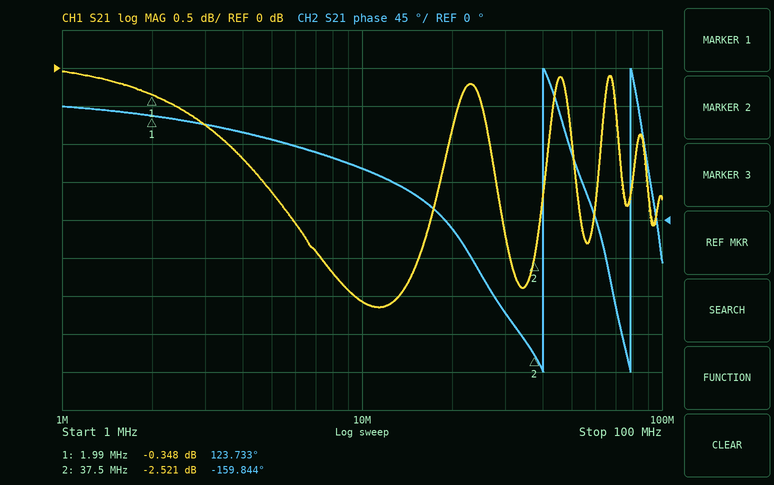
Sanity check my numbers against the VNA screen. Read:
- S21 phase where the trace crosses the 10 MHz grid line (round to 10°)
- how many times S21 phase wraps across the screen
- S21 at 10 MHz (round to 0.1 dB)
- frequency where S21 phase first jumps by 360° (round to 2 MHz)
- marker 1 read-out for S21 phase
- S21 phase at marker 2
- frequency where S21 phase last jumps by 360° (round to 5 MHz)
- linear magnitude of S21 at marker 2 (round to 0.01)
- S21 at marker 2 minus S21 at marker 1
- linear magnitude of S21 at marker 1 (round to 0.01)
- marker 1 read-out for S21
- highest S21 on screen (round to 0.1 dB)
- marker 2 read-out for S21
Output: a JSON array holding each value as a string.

["60°", "2", "-3.1 dB", "40 MHz", "123.733°", "-159.844°", "80 MHz", "0.75", "-2.173 dB", "0.96", "-0.348 dB", "0.0 dB", "-2.521 dB"]
